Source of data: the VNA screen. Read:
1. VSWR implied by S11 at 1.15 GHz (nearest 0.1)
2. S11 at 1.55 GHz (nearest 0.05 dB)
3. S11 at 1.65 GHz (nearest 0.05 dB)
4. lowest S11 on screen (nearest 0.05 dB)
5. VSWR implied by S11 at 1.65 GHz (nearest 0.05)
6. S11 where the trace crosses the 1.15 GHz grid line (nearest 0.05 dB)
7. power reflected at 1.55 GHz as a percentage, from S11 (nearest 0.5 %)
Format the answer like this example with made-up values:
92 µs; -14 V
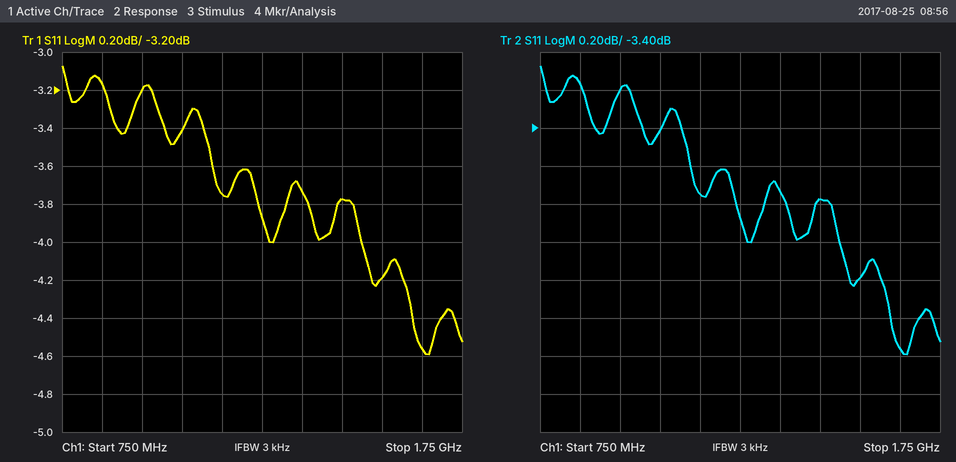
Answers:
4.7; -4.20 dB; -4.55 dB; -4.60 dB; 3.90; -3.75 dB; 38.0 %
